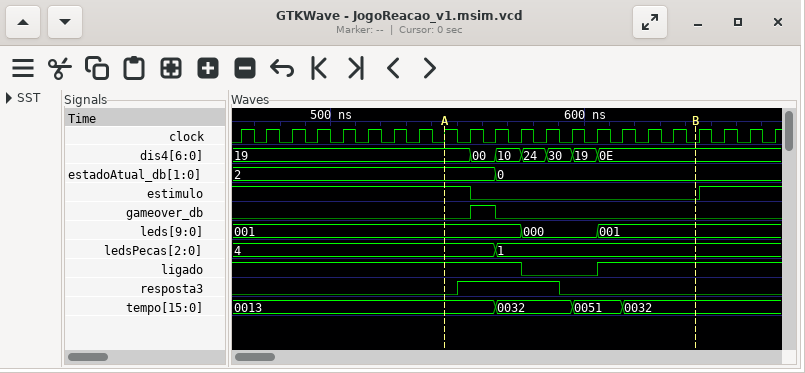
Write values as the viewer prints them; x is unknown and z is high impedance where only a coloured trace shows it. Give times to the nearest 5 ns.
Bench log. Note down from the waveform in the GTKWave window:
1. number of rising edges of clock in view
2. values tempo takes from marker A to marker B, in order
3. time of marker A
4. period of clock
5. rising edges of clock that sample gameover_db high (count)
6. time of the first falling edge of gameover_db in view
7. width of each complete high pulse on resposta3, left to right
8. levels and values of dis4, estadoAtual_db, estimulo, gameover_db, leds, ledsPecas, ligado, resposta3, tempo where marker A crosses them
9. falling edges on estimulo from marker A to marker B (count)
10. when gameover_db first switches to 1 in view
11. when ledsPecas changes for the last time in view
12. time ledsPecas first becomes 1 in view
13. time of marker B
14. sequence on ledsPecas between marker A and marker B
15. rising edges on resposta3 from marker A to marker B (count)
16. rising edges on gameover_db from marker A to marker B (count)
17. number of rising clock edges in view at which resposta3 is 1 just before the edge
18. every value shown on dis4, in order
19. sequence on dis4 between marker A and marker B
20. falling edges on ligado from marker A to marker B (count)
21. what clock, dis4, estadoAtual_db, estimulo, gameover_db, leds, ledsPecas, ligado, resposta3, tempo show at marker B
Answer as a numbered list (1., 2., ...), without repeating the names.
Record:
1. 22
2. 0013, 0032, 0051, 0032
3. 545 ns
4. 10 ns
5. 1
6. 565 ns
7. 40 ns
8. dis4=19, estadoAtual_db=2, estimulo=1, gameover_db=0, leds=001, ledsPecas=4, ligado=1, resposta3=0, tempo=0013
9. 1
10. 555 ns
11. 565 ns
12. 565 ns
13. 645 ns
14. 4, 1
15. 1
16. 1
17. 4
18. 19, 00, 10, 24, 30, 19, 0E
19. 19, 00, 10, 24, 30, 19, 0E
20. 1
21. clock=0, dis4=0E, estadoAtual_db=0, estimulo=0, gameover_db=0, leds=001, ledsPecas=1, ligado=1, resposta3=0, tempo=0032
